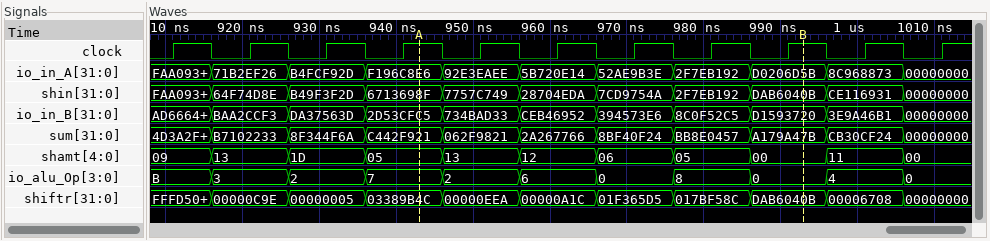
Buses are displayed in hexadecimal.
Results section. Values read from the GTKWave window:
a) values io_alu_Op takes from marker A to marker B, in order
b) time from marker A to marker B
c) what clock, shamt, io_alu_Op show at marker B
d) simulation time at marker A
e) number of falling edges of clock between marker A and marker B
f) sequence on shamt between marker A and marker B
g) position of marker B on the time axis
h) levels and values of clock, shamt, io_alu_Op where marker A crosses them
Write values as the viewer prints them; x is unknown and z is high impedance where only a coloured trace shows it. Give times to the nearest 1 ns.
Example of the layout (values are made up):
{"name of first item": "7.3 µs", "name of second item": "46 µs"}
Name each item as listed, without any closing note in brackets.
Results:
{"values io_alu_Op takes from marker A to marker B, in order": "7, 2, 6, 0, 8, 0", "time from marker A to marker B": "50 ns", "what clock, shamt, io_alu_Op show at marker B": "clock=1, shamt=00, io_alu_Op=0", "simulation time at marker A": "943 ns", "number of falling edges of clock between marker A and marker B": "5", "sequence on shamt between marker A and marker B": "05, 13, 12, 06, 05, 00", "position of marker B on the time axis": "993 ns", "levels and values of clock, shamt, io_alu_Op where marker A crosses them": "clock=1, shamt=05, io_alu_Op=7"}
